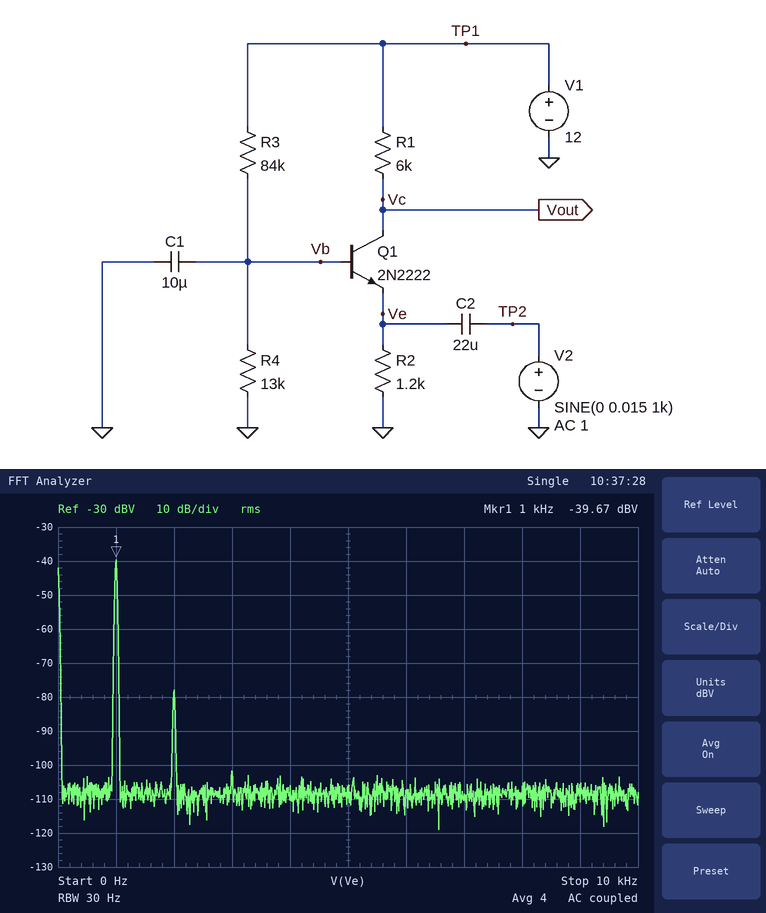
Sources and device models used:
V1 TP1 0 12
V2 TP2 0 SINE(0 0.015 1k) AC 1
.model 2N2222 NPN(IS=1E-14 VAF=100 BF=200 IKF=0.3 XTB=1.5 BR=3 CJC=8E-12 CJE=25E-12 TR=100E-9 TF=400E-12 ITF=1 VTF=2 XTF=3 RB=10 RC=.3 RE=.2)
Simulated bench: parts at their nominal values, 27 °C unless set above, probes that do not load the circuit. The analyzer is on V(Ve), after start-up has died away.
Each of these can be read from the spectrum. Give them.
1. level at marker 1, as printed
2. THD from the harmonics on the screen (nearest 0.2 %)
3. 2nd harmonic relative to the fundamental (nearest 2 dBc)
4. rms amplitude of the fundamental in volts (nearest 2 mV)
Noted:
-39.67 dBV
1.2 %
-38 dBc
10 mV
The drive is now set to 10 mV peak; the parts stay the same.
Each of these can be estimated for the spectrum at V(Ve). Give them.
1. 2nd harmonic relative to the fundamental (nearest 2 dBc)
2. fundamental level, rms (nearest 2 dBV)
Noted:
-42 dBc
-44 dBV
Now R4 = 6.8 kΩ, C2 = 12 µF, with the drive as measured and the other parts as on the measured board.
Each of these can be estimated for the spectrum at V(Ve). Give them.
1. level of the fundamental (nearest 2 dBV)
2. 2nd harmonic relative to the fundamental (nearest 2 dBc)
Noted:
-40 dBV
-42 dBc
